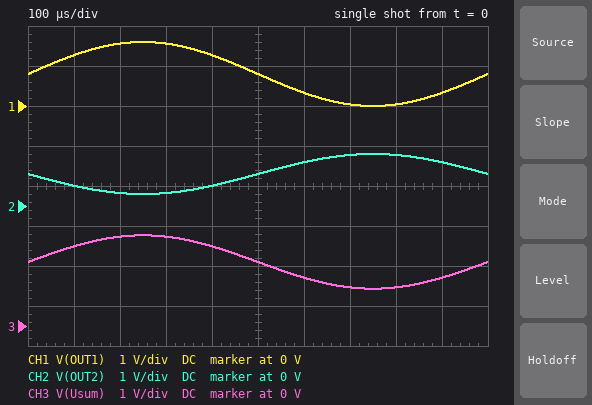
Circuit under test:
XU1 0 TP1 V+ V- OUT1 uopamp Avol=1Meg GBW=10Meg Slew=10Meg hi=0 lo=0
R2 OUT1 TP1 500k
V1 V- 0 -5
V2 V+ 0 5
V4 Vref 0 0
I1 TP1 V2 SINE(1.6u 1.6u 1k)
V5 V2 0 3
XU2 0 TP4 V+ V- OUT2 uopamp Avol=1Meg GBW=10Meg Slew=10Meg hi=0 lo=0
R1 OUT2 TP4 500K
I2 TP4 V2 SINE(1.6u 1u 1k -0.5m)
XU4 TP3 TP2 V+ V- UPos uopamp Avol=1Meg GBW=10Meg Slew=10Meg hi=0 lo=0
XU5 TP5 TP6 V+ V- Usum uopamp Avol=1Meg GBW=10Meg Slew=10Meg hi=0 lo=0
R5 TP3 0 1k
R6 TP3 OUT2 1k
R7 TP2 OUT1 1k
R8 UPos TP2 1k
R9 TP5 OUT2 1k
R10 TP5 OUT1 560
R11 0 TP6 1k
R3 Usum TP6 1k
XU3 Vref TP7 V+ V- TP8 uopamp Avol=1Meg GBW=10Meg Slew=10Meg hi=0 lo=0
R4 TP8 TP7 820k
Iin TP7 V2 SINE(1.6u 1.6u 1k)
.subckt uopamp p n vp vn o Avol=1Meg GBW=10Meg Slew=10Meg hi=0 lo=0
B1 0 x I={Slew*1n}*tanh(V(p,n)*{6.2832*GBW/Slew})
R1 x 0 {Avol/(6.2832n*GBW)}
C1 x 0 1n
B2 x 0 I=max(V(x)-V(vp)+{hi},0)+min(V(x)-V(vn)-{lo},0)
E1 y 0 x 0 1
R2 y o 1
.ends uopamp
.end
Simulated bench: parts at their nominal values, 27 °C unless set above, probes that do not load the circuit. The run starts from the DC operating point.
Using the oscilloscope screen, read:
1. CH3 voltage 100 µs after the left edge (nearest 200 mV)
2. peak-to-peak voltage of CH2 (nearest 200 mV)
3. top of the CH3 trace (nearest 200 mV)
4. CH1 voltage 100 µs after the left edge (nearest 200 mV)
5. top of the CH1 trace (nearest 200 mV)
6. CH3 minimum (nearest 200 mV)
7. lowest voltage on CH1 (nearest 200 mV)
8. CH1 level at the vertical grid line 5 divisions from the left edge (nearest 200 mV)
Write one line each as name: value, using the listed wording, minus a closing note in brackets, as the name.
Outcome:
CH3 voltage 100 µs after the left edge: 2.0 V
peak-to-peak voltage of CH2: 1.0 V
top of the CH3 trace: 2.2 V
CH1 voltage 100 µs after the left edge: 1.2 V
top of the CH1 trace: 1.6 V
CH3 minimum: 1.0 V
lowest voltage on CH1: 0 V
CH1 level at the vertical grid line 5 divisions from the left edge: 800 mV
